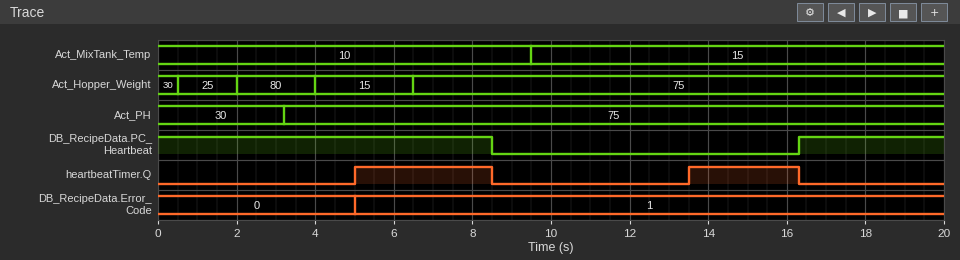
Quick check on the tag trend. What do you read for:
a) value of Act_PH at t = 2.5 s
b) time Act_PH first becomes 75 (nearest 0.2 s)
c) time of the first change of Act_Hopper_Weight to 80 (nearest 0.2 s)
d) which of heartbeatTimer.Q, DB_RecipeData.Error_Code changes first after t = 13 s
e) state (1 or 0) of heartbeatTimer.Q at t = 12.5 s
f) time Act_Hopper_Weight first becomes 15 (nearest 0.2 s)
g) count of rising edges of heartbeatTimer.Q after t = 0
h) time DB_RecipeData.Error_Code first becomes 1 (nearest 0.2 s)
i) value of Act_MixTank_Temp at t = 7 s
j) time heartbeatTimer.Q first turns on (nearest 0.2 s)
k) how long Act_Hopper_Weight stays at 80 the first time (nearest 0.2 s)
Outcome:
30
3.2 s
2.0 s
heartbeatTimer.Q
0
4.0 s
2
5.0 s
10
5.0 s
2.0 s
